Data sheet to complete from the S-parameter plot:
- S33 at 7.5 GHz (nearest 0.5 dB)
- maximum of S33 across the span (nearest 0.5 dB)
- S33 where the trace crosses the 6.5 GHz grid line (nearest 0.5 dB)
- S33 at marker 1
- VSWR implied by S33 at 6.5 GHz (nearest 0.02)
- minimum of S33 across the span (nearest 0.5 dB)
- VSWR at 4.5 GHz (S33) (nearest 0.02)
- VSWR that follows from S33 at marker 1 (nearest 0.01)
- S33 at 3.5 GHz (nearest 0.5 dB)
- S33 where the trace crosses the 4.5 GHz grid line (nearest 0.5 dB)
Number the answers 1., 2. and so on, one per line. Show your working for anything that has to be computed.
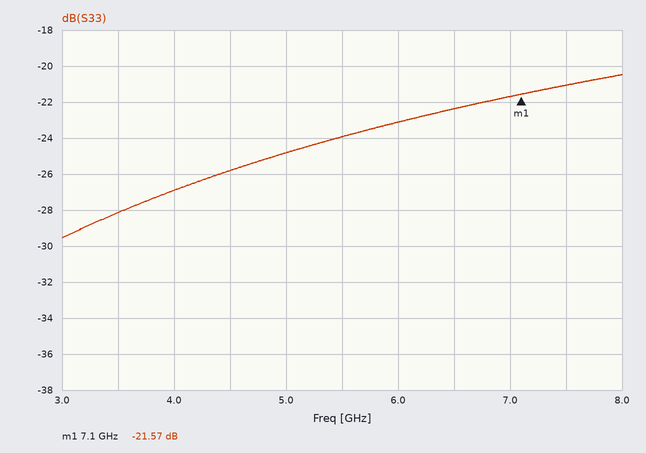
1. -21.0 dB
2. -20.5 dB
3. -22.5 dB
4. -21.57 dB
5. |Γ| = 10^(-22.5/20) = 0.0750; VSWR = (1 + 0.0750)/(1 − 0.0750) ≈ 1.16
6. -29.5 dB
7. |Γ| = 10^(-26/20) = 0.0501; VSWR = (1 + 0.0501)/(1 − 0.0501) ≈ 1.11, so 1.10 to the nearest 0.02
8. (1 + 0.0835)/(1 − 0.0835) ≈ 1.18
9. -28.0 dB
10. -26.0 dB
